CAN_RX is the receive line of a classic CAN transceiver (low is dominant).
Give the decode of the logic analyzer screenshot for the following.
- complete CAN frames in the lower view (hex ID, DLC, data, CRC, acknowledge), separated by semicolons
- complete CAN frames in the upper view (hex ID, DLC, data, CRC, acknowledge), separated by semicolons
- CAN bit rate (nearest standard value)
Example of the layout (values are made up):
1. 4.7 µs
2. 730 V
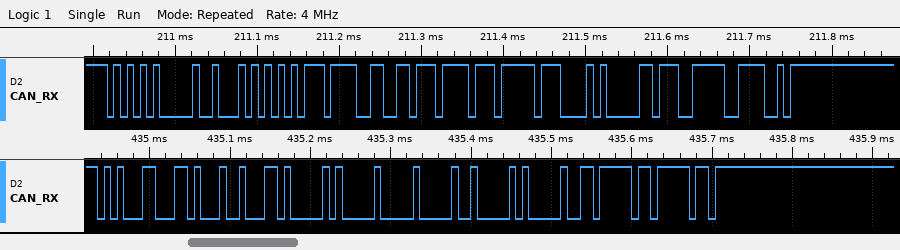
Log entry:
1. ID 14611234, DLC 4, data 00 01 02 03, CRC 3FBF, ACK
2. ID 550, DLC 8, data AA BB CC DD EE FF 0A 0B, CRC 4FBC, ACK
3. 125 kbit/s
